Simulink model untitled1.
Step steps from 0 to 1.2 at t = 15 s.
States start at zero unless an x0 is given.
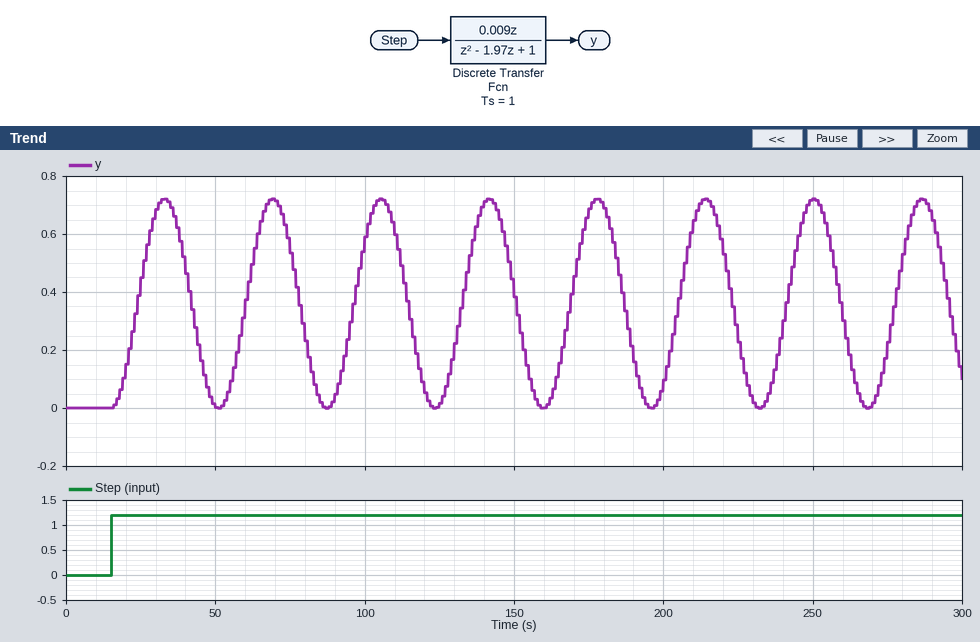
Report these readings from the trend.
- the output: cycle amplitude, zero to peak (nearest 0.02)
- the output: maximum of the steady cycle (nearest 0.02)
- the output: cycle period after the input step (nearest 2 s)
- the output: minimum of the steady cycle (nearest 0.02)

0.36
0.72
36 s
0.00
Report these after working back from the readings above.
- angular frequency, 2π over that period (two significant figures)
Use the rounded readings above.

0.17 rad/s
